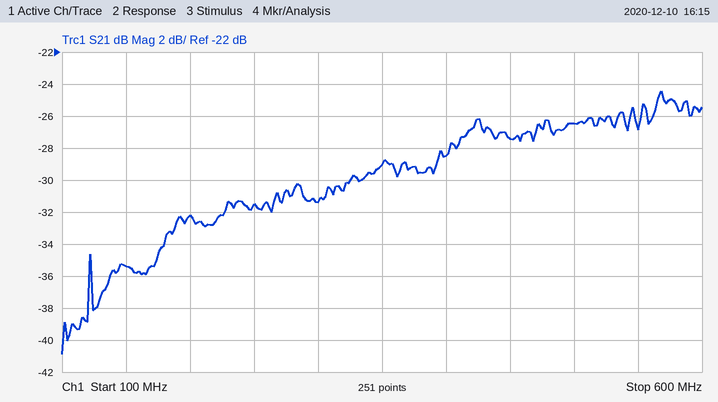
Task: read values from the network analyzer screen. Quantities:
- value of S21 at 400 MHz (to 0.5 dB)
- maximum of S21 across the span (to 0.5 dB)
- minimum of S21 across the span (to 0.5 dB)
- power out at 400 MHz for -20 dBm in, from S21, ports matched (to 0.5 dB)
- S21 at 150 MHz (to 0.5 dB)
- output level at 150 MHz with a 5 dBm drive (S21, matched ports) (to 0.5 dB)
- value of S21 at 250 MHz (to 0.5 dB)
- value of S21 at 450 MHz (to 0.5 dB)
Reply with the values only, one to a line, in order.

-28.5 dB
-24.5 dB
-41.0 dB
-48.5 dBm
-35.5 dB
-30.5 dBm
-31.5 dB
-27.5 dB
